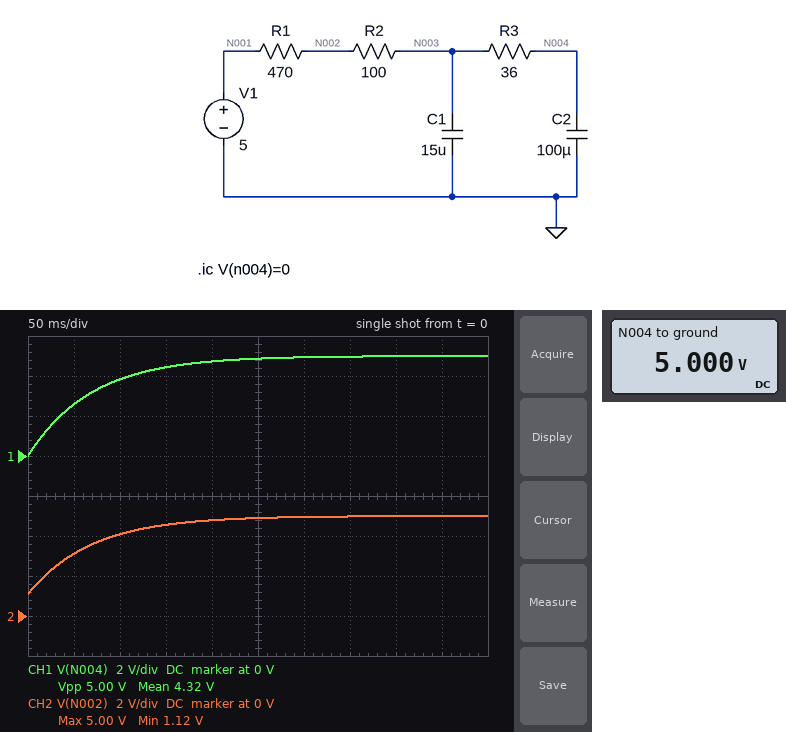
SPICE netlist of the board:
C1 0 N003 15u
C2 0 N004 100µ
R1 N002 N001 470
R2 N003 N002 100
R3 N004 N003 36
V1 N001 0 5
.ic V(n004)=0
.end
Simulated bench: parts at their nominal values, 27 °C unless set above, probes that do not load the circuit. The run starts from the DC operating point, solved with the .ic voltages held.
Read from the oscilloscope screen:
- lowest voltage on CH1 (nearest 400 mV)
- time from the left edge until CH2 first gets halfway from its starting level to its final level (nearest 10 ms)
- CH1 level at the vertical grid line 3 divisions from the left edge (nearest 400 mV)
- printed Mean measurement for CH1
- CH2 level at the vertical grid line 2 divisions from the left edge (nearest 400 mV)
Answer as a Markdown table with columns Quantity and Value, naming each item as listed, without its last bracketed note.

| Quantity | Value |
|---|---|
| lowest voltage on CH1 | 0 V |
| time from the left edge until CH2 first gets halfway from its starting level to its final level | 50 ms |
| CH1 level at the vertical grid line 3 divisions from the left edge | 4.4 V |
| printed Mean measurement for CH1 | 4.32 V |
| CH2 level at the vertical grid line 2 divisions from the left edge | 4.0 V |
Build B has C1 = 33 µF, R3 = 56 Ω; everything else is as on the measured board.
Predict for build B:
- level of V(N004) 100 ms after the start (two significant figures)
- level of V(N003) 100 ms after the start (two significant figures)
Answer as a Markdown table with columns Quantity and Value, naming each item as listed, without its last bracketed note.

| Quantity | Value |
|---|---|
| level of V(N004) 100 ms after the start | 3.6 V |
| level of V(N003) 100 ms after the start | 3.7 V |
